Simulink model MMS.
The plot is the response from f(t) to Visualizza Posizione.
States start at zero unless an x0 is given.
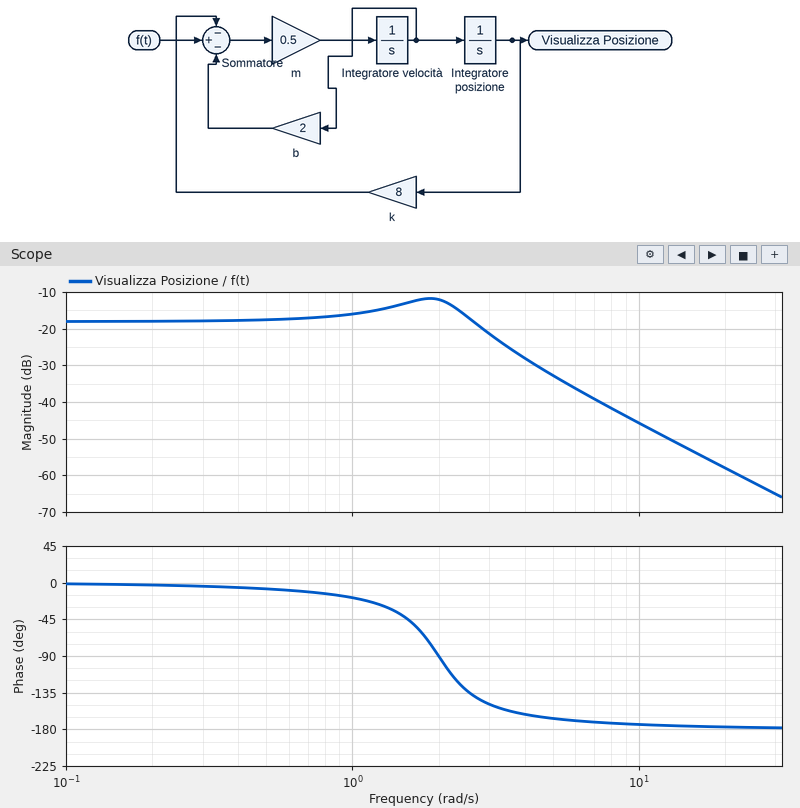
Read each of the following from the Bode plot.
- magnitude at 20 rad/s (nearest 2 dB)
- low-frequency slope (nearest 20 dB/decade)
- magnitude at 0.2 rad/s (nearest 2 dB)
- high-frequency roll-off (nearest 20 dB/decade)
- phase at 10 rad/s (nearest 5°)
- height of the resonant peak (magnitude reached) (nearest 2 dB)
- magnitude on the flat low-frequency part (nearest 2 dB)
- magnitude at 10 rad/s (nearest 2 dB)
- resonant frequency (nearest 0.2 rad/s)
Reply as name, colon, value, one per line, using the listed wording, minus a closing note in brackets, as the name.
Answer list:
magnitude at 20 rad/s: -58 dB
low-frequency slope: 0 dB/decade
magnitude at 0.2 rad/s: -18 dB
high-frequency roll-off: -40 dB/decade
phase at 10 rad/s: -175°
height of the resonant peak (magnitude reached): -12 dB
magnitude on the flat low-frequency part: -18 dB
magnitude at 10 rad/s: -46 dB
resonant frequency: 1.8 rad/s
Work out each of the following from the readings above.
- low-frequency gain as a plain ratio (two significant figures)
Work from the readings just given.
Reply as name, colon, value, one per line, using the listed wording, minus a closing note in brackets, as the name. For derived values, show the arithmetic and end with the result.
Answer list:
low-frequency gain as a plain ratio: 10^(-18 / 20) = 0.13
